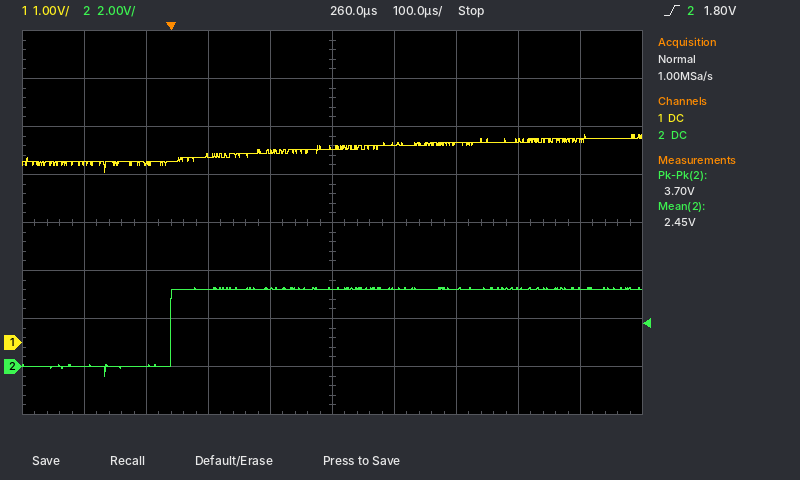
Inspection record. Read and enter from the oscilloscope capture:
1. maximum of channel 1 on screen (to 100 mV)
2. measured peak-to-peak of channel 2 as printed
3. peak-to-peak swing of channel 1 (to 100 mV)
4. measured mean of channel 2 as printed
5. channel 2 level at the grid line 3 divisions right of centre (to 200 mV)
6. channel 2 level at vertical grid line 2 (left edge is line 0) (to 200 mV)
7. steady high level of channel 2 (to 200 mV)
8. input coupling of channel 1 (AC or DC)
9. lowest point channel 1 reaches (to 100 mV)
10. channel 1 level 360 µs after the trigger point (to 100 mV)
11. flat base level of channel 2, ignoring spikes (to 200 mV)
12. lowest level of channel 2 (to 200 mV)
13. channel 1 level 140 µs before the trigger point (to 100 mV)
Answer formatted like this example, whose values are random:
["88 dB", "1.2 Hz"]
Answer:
["4.3 V", "3.70 V", "800 mV", "2.45 V", "3.2 V", "0.0 V", "3.2 V", "DC", "3.5 V", "4.1 V", "0.0 V", "-400 mV", "3.7 V"]
